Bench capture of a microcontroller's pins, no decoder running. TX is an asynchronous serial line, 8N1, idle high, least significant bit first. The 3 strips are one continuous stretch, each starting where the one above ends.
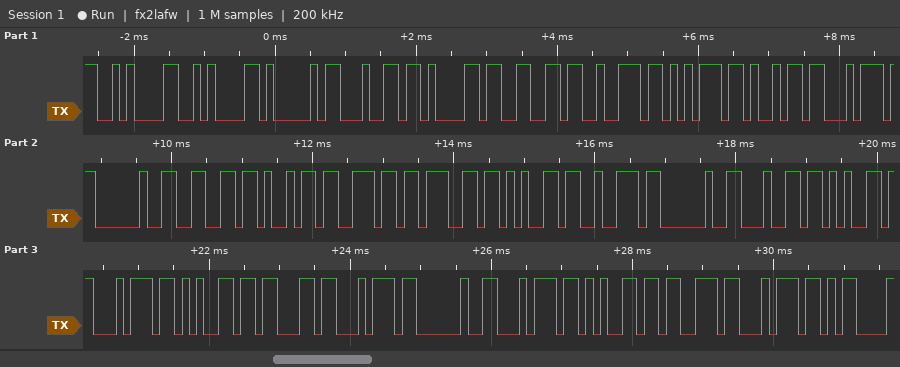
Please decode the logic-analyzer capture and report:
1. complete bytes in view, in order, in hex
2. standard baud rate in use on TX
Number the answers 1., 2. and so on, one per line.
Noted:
1. 0x0A 0x0A 0x41 0x64 0x61 0x66 0x72 0x75 0x69 0x74 0x20 0x66 0x69 0x6E 0x67 0x65 0x72 0x20 0x64 0x65 0x74 0x65 0x63 0x74 0x20 0x74 0x65 0x73 0x74 0x0D
2. 9600 baud
